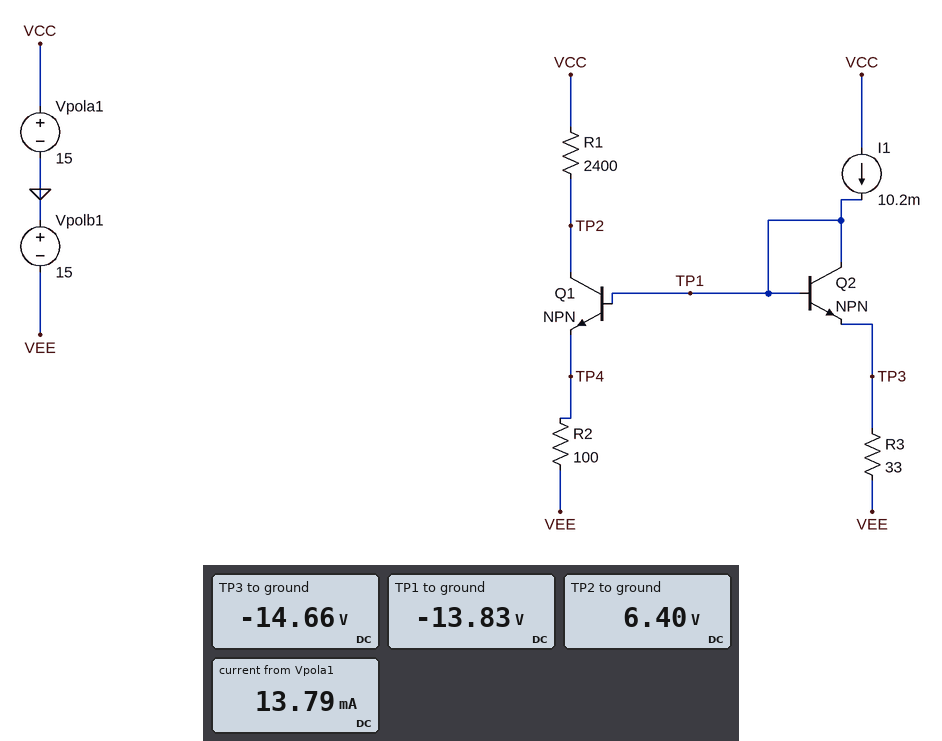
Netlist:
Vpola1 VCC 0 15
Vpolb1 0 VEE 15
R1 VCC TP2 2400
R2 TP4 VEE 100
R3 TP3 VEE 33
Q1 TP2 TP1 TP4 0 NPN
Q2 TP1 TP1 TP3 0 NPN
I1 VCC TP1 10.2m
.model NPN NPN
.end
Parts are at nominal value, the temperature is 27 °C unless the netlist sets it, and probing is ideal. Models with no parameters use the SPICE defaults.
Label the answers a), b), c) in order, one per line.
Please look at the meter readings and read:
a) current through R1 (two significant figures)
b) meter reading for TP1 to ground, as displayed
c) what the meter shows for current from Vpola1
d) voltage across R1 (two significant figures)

a) 3.6 mA
b) -13.83 V
c) 13.79 mA
d) 8.6 V
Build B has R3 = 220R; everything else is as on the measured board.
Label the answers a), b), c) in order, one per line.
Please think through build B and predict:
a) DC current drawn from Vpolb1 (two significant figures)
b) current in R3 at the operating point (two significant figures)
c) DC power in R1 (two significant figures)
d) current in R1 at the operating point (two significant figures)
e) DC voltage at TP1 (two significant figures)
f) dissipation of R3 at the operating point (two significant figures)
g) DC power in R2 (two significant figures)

a) 22 mA
b) 7.0 mA
c) 340 mW
d) 12 mA
e) -13 V
f) 11 mW
g) 23 mW
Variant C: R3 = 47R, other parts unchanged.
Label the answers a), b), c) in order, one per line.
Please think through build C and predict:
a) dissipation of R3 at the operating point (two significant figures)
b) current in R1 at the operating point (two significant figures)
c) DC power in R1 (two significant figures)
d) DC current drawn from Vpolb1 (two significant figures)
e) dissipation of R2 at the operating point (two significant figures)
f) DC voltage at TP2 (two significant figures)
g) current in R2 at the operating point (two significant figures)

a) 4.8 mW
b) 4.9 mA
c) 58 mW
d) 15 mA
e) 2.5 mW
f) 3.2 V
g) 5.0 mA
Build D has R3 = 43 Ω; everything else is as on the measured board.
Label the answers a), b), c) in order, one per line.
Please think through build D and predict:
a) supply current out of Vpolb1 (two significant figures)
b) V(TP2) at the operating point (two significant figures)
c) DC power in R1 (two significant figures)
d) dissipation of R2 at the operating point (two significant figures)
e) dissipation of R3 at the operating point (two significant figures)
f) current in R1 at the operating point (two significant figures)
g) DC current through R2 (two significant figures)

a) 15 mA
b) 4.1 V
c) 49 mW
d) 2.1 mW
e) 4.4 mW
f) 4.5 mA
g) 4.6 mA
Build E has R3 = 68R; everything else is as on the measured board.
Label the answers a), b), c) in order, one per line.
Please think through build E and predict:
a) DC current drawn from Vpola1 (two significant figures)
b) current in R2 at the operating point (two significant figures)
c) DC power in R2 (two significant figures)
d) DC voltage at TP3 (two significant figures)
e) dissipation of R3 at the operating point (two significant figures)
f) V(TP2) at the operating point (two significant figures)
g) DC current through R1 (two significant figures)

a) 17 mA
b) 7.0 mA
c) 4.9 mW
d) -14 V
e) 7.0 mW
f) -1.6 V
g) 6.9 mA
